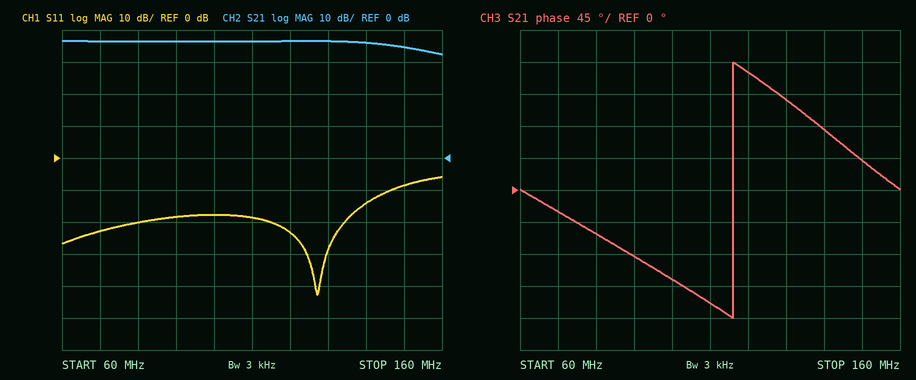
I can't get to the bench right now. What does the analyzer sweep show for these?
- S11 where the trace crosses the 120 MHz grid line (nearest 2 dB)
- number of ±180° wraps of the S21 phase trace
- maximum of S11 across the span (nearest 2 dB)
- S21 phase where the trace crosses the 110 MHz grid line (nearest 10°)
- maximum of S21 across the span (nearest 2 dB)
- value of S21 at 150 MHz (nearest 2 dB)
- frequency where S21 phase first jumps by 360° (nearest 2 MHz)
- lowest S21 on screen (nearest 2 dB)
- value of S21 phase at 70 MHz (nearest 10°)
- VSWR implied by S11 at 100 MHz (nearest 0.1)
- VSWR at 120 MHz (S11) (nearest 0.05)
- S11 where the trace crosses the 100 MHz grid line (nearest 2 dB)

-24 dB
1
-6 dB
-160°
36 dB
34 dB
116 MHz
32 dB
-30°
1.3
1.15
-18 dB
